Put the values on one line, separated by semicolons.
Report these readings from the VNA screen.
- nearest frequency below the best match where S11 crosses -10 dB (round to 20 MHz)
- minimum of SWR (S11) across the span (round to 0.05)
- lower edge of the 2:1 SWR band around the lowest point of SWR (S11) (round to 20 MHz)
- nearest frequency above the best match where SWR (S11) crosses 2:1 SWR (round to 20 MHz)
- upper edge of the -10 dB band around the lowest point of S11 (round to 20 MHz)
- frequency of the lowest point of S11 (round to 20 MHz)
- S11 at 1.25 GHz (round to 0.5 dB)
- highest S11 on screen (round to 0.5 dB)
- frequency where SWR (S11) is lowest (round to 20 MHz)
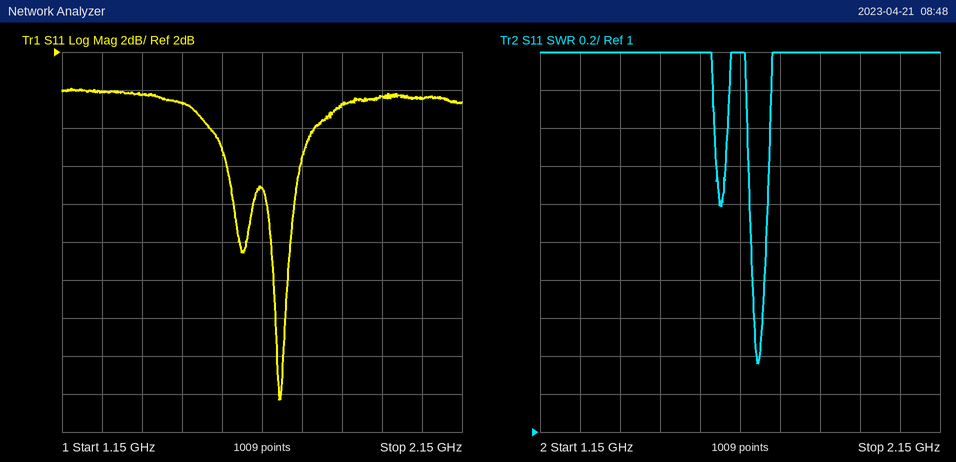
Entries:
1.68 GHz; 1.35; 1.68 GHz; 1.72 GHz; 1.72 GHz; 1.70 GHz; 0.0 dB; 0.0 dB; 1.70 GHz
